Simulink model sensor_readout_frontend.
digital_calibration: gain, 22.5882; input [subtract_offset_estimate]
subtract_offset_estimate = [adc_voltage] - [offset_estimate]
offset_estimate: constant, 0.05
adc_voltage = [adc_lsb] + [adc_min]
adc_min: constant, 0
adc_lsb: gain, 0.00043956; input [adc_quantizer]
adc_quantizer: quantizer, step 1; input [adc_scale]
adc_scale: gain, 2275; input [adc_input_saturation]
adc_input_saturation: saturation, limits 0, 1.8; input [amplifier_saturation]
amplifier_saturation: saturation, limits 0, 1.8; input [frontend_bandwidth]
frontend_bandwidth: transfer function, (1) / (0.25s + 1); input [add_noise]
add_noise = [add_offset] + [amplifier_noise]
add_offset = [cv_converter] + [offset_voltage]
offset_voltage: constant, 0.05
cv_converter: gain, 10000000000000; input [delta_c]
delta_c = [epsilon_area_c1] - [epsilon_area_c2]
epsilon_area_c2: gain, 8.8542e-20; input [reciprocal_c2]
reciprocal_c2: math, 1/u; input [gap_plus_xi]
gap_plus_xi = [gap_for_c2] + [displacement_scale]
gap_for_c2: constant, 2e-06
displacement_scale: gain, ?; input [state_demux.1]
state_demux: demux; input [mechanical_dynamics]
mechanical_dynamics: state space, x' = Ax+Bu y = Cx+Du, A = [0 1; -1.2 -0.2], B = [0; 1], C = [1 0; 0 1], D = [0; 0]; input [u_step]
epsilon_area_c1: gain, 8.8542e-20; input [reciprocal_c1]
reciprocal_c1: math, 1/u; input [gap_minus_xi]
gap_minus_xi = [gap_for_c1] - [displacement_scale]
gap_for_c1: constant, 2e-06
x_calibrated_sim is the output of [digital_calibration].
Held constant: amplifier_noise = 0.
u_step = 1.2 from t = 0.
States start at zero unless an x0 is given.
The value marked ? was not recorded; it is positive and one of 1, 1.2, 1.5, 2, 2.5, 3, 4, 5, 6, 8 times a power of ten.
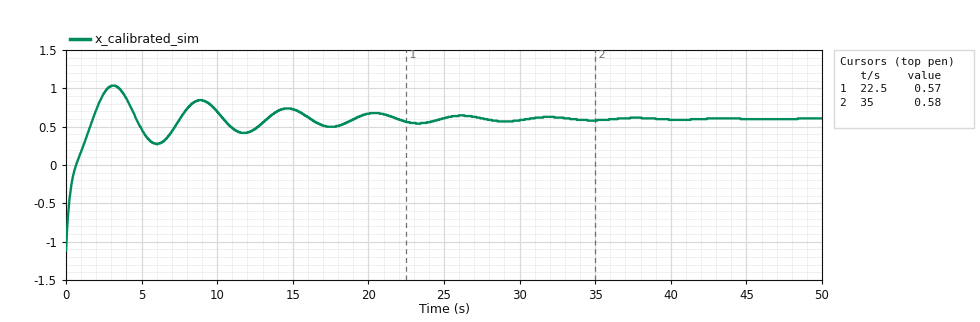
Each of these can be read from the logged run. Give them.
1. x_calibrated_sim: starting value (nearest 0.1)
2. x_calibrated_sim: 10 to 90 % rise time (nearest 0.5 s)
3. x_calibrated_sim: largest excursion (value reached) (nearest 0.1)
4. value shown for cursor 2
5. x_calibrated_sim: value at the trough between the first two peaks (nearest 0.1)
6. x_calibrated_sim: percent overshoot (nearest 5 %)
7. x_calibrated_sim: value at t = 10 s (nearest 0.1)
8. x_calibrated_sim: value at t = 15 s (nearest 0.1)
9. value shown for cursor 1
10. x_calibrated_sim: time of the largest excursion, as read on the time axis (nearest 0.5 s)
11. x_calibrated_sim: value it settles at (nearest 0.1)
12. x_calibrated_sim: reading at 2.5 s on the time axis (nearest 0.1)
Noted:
-1.1
1.5 s
1.0
0.58
0.3
25 %
0.7
0.7
0.57
3.0 s
0.6
0.9
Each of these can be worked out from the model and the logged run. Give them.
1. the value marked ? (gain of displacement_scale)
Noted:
6e-08
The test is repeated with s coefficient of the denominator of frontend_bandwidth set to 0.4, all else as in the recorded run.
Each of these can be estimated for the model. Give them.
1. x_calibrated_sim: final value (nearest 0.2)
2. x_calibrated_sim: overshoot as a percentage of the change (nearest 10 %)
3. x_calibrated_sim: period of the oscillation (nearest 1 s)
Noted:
0.6
20 %
6 s
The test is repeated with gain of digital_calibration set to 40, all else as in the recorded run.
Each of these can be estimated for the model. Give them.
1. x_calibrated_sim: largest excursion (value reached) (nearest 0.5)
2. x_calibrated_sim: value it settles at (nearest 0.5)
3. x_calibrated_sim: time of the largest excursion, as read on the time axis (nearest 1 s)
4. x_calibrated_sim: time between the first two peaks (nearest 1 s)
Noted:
2.0
1.0
3 s
6 s
